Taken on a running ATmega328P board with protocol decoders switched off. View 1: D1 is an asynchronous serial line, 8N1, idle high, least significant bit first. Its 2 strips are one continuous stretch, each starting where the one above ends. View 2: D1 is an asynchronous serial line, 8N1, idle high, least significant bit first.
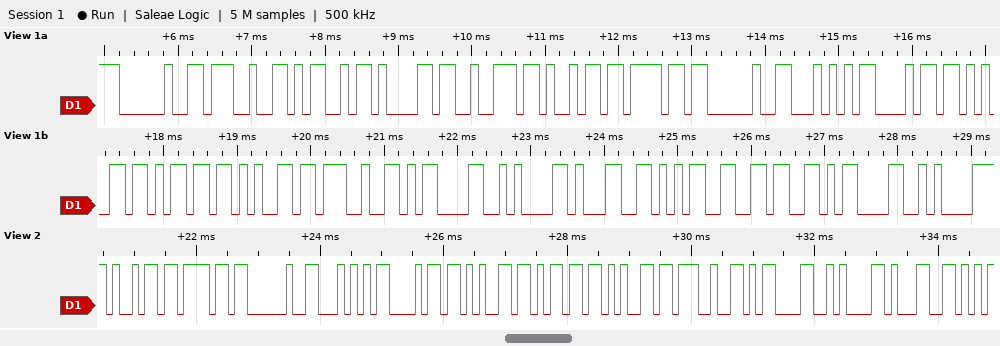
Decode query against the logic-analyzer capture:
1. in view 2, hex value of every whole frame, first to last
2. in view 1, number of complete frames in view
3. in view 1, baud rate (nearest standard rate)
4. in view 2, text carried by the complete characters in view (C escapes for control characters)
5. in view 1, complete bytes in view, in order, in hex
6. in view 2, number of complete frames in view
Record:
0x69 0x6F 0x20 0x54 0x68 0x65 0x6D 0x65 0x27 0x0D 0x0A 0x31
21
9600 baud
"io Theme'\r\n1"
0x20 0x27 0x4D 0x61 0x72 0x69 0x6F 0x20 0x54 0x68 0x65 0x6D 0x65 0x27 0x0D 0x0A 0x31 0x35 0x36 0x0D 0x0A
12
